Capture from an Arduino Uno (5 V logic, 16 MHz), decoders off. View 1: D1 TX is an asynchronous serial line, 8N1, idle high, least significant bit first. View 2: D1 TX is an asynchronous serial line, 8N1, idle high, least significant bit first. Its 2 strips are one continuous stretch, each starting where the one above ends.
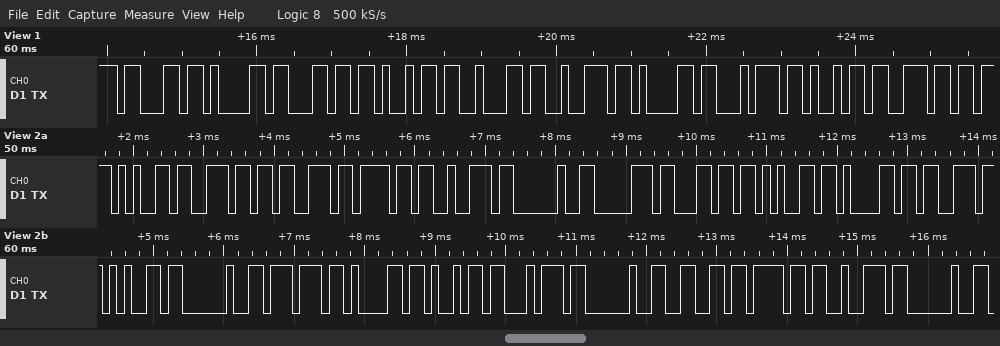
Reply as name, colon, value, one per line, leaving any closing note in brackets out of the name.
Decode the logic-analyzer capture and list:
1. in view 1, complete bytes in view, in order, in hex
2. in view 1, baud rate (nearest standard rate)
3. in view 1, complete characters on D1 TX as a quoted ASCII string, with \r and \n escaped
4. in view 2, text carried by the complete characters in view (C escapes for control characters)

in view 1, complete bytes in view, in order, in hex: 0x63 0x61 0x6C 0x69 0x62 0x72 0x61 0x74 0x69 0x6E
in view 1, baud rate: 9600 baud
in view 1, complete characters on D1 TX as a quoted ASCII string, with \r and \n escaped: "calibratin"
in view 2, text carried by the complete characters in view: "ensor please wait for "
